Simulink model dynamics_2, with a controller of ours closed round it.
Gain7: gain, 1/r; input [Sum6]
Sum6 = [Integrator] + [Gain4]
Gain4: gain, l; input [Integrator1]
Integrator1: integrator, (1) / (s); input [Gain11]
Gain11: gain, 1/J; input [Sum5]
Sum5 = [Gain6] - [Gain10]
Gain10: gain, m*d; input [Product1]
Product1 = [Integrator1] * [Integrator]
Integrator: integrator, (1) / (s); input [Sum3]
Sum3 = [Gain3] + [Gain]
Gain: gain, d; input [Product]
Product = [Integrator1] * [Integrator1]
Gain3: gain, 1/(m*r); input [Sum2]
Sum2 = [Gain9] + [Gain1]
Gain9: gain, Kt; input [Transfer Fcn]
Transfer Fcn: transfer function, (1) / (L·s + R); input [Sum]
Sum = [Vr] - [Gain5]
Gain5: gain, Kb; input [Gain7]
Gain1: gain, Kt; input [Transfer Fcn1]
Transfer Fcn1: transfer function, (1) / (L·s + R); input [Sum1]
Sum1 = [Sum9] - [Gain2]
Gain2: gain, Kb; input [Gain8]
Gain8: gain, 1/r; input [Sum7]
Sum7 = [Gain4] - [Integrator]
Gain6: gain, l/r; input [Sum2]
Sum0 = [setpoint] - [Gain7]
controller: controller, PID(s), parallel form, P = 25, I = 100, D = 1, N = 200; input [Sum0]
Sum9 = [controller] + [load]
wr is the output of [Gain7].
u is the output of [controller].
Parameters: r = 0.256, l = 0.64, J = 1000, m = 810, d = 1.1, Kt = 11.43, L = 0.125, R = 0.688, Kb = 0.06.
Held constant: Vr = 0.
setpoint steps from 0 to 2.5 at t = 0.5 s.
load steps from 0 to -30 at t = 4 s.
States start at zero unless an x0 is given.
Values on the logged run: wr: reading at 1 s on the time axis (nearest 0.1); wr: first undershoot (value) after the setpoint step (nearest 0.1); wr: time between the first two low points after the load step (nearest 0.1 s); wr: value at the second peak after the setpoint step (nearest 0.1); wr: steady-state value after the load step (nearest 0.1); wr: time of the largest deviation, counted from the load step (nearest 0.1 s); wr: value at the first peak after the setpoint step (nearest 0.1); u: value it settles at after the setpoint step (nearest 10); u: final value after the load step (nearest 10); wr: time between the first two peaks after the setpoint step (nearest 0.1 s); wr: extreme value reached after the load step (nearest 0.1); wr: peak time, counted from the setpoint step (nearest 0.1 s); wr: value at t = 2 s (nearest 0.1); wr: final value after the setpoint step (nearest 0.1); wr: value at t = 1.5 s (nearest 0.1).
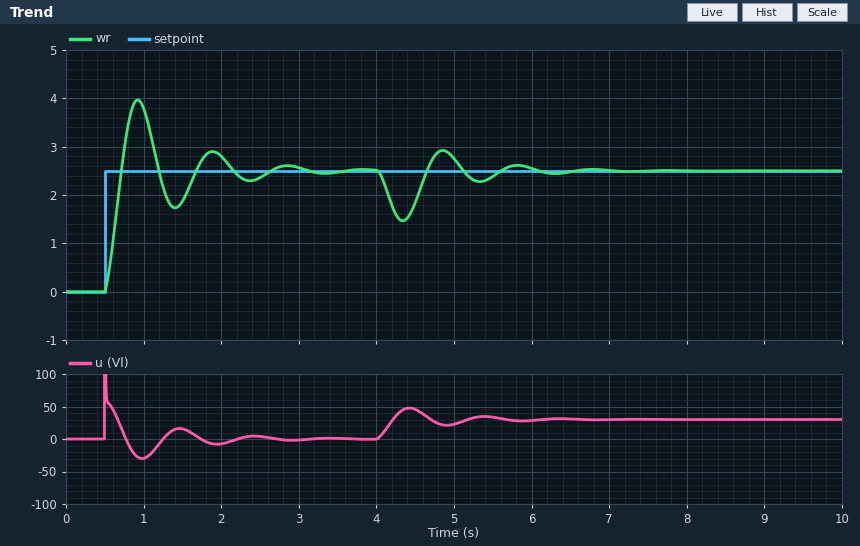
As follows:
3.8
1.7
1.0 s
2.9
2.5
0.3 s
4.0
0
30
1.0 s
1.5
0.4 s
2.8
2.5
1.9
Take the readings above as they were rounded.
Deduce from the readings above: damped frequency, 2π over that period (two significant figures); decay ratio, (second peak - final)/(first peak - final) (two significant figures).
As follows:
6.3 rad/s
0.27
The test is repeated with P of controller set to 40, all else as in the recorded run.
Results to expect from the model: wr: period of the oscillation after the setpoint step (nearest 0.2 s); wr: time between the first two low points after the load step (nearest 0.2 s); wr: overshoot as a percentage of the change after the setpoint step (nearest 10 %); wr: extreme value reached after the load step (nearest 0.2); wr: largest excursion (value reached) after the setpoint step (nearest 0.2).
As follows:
0.8 s
0.8 s
50 %
1.8
3.8
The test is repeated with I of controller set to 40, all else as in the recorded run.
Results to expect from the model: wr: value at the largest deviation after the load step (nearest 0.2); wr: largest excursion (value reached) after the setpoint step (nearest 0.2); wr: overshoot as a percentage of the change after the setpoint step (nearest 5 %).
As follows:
1.4
3.4
35 %
